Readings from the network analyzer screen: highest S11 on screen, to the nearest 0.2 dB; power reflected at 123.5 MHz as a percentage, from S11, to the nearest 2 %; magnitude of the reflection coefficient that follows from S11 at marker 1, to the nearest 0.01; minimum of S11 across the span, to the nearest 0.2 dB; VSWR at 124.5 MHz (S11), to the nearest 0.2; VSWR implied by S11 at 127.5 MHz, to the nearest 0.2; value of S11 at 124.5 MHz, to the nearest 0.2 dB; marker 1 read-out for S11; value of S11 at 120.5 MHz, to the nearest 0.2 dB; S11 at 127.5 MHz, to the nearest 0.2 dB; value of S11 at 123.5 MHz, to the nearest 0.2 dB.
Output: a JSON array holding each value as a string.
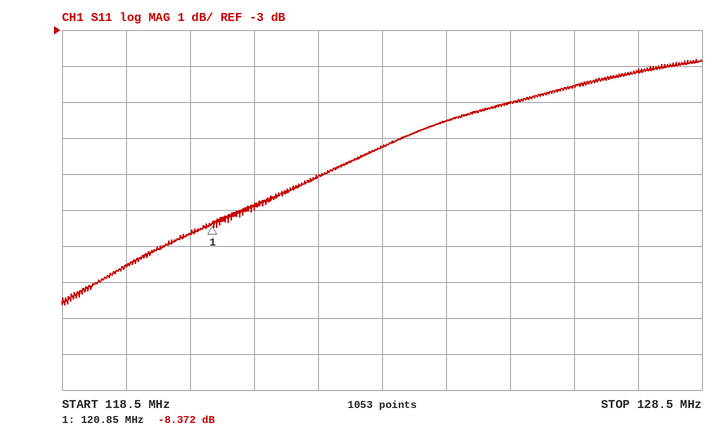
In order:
["-3.8 dB", "24 %", "0.38", "-10.6 dB", "3.2", "4.2", "-5.6 dB", "-8.372 dB", "-8.6 dB", "-4.2 dB", "-6.2 dB"]
